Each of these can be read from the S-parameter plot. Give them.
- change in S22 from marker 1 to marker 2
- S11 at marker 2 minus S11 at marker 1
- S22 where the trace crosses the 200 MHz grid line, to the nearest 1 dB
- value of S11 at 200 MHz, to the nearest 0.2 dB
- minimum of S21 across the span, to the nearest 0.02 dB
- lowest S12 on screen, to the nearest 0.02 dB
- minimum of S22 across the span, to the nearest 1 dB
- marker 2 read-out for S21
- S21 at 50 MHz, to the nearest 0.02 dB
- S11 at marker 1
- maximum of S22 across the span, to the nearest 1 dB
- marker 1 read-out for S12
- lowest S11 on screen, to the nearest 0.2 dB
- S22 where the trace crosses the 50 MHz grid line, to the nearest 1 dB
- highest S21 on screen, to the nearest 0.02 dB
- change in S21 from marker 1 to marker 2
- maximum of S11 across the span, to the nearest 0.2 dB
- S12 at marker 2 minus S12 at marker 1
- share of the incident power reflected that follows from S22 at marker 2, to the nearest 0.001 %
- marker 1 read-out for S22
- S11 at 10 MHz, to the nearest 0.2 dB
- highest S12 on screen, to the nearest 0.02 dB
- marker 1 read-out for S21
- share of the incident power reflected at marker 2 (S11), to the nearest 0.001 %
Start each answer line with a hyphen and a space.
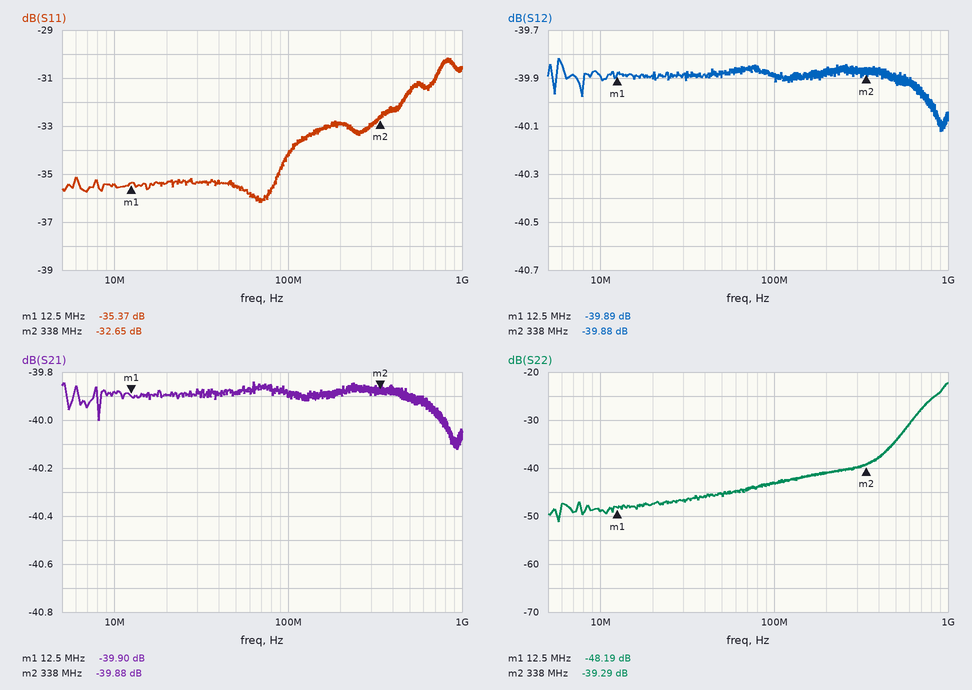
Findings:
- 8.90 dB
- 2.72 dB
- -41 dB
- -32.8 dB
- -40.12 dB
- -40.12 dB
- -51 dB
- -39.88 dB
- -39.88 dB
- -35.37 dB
- -22 dB
- -39.89 dB
- -36.2 dB
- -45 dB
- -39.84 dB
- 0.02 dB
- -30.2 dB
- 0.01 dB
- 0.012 %
- -48.19 dB
- -35.4 dB
- -39.82 dB
- -39.90 dB
- 0.054 %
